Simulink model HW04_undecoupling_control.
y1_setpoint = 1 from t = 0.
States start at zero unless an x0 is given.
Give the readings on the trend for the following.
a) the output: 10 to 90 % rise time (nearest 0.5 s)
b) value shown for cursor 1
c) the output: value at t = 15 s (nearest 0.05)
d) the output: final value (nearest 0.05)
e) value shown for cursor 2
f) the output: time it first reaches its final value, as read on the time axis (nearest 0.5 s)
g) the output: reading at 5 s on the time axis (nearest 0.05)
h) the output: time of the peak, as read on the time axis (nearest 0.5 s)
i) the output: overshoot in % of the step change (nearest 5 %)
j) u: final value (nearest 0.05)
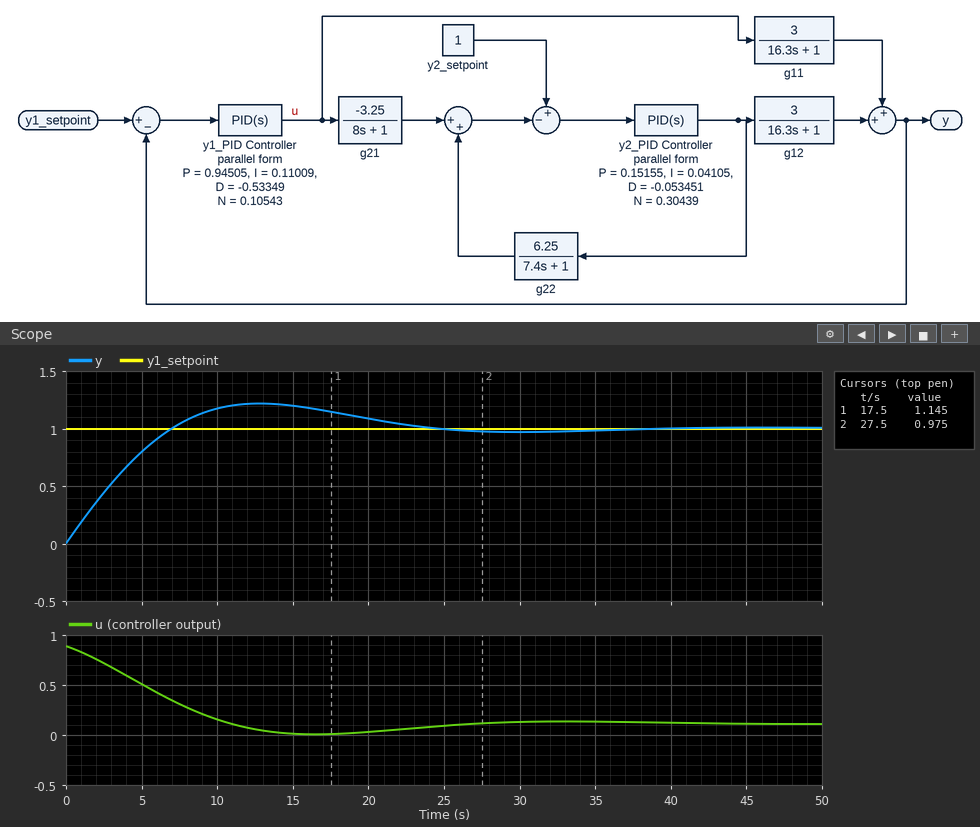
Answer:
5.5 s
1.145
1.20
1.00
0.975
7.0 s
0.80
13.0 s
20 %
0.10
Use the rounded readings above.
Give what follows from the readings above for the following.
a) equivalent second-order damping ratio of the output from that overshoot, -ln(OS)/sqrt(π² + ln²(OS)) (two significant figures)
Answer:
0.46
